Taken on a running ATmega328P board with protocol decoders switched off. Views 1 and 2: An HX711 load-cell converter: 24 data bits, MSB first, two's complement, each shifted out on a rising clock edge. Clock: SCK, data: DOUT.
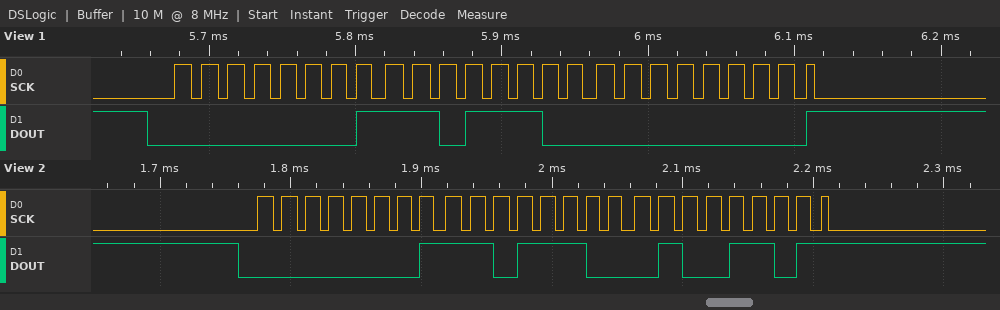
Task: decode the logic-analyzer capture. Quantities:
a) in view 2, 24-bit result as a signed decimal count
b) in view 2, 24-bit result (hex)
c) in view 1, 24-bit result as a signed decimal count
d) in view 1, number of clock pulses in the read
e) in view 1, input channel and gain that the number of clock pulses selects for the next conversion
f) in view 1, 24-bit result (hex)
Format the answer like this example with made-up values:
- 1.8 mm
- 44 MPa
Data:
- 121933
- 0x01DC4D
- 121856
- 25
- channel A, gain 128
- 0x01DC00
